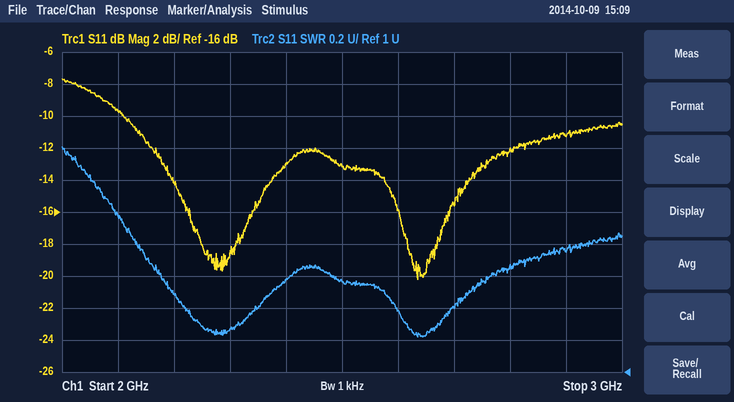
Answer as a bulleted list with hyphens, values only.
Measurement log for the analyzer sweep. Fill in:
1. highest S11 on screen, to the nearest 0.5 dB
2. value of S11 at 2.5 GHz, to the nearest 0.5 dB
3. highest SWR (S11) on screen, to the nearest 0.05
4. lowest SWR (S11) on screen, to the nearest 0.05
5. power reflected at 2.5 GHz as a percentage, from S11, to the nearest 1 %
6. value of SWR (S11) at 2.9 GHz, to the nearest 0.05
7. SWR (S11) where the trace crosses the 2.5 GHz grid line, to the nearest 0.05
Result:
- -7.5 dB
- -13.0 dB
- 2.40
- 1.20
- 5 %
- 1.75
- 1.55
